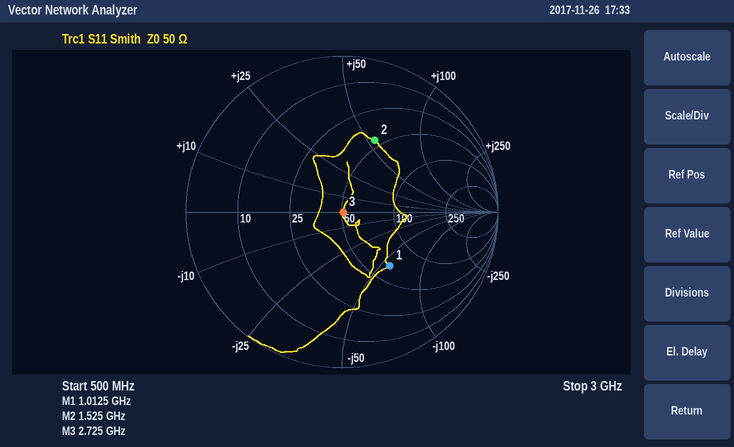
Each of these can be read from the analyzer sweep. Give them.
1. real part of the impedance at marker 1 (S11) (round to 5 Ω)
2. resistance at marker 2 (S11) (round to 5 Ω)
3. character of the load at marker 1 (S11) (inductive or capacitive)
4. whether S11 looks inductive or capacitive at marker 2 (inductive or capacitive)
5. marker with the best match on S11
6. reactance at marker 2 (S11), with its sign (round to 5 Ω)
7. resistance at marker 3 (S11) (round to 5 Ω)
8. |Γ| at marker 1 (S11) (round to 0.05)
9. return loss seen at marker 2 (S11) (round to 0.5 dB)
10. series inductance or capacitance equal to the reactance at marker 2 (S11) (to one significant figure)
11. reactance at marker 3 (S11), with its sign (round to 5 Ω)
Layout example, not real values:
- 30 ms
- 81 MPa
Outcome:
- 65 Ω
- 45 Ω
- capacitive
- inductive
- marker 3
- +55 Ω
- 50 Ω
- 0.45
- 6.0 dB
- 6 nH
- 0 Ω
